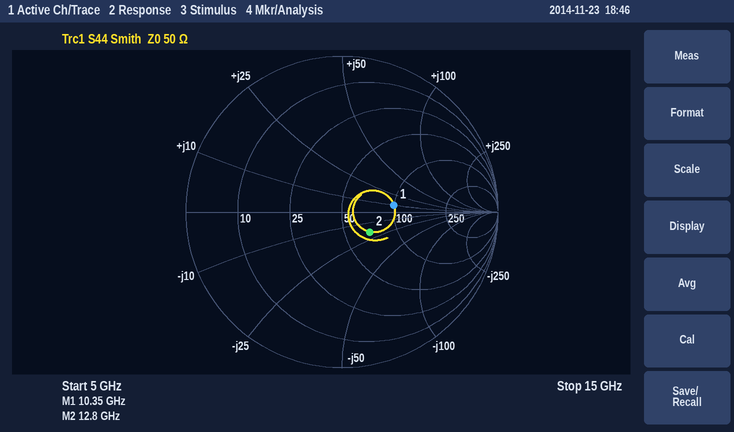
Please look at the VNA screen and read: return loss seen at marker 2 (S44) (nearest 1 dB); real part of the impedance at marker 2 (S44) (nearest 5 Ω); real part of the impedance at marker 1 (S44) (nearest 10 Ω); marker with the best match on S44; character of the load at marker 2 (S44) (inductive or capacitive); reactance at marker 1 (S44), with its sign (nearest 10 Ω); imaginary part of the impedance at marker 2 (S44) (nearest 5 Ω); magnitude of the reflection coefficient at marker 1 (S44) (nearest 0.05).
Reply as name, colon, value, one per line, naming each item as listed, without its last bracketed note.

return loss seen at marker 2 (S44): 13 dB
real part of the impedance at marker 2 (S44): 70 Ω
real part of the impedance at marker 1 (S44): 100 Ω
marker with the best match on S44: marker 2
character of the load at marker 2 (S44): capacitive
reactance at marker 1 (S44), with its sign: +10 Ω
imaginary part of the impedance at marker 2 (S44): -20 Ω
magnitude of the reflection coefficient at marker 1 (S44): 0.35
